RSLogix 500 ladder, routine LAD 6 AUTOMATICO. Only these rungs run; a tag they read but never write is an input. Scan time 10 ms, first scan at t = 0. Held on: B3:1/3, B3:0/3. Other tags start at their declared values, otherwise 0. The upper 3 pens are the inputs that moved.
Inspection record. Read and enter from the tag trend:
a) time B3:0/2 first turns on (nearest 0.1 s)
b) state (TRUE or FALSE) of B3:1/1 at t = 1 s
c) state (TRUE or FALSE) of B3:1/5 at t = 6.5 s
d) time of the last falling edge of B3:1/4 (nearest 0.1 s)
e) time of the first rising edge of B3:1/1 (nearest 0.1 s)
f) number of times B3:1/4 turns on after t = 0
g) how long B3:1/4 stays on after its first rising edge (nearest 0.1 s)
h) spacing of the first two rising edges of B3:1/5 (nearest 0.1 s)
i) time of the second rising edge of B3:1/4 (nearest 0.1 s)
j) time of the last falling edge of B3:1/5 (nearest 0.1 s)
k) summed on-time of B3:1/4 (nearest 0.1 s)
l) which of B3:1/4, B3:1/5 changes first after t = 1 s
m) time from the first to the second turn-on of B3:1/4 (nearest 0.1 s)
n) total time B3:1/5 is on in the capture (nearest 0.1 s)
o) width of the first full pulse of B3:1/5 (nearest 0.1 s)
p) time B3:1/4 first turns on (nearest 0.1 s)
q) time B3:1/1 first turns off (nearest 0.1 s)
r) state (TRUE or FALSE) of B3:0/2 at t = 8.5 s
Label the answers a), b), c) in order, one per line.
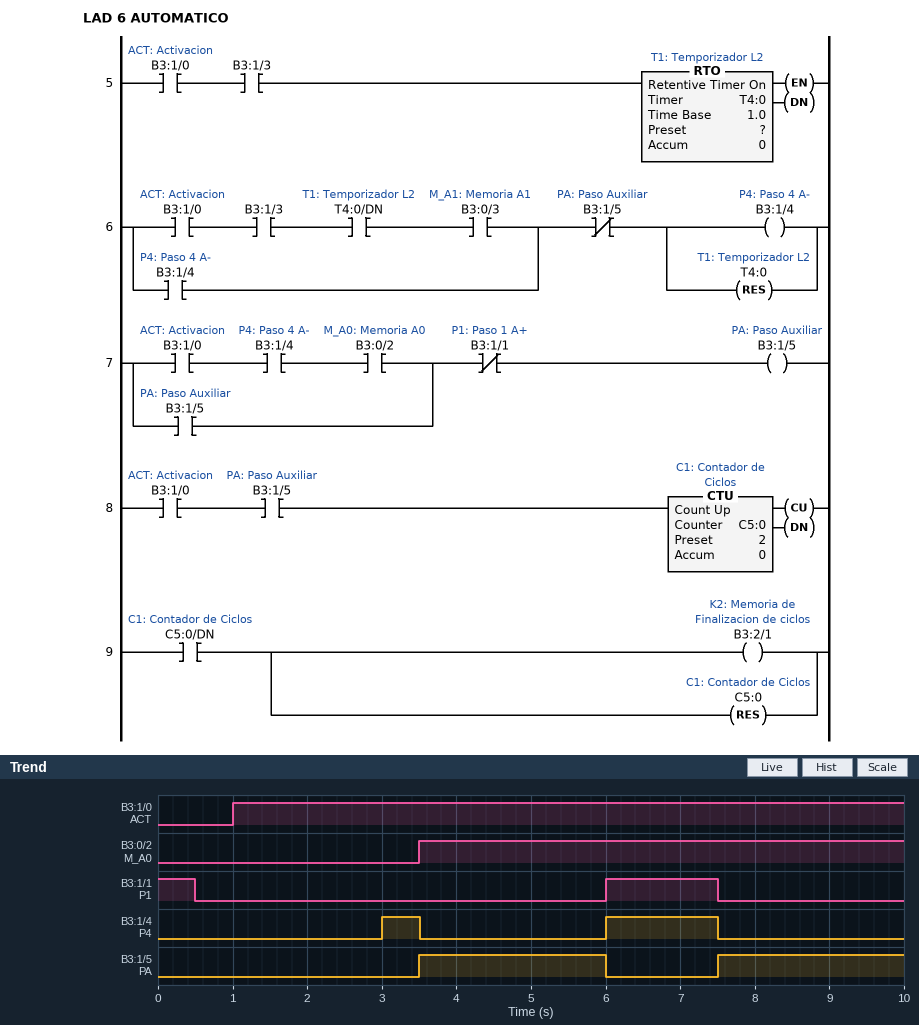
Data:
a) 3.5 s
b) FALSE
c) FALSE
d) 7.5 s
e) 6.0 s
f) 2
g) 0.5 s
h) 4.0 s
i) 6.0 s
j) 6.0 s
k) 2.0 s
l) B3:1/4
m) 3.0 s
n) 5.0 s
o) 2.5 s
p) 3.0 s
q) 0.5 s
r) TRUE
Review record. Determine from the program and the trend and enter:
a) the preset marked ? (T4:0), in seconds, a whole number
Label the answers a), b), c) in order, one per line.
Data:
a) 2 s
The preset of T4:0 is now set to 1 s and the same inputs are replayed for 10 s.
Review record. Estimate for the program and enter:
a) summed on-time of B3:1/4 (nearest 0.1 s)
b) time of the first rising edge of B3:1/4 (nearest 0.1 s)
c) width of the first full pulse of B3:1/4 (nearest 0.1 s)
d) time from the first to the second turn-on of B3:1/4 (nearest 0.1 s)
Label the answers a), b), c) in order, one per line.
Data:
a) 3.0 s
b) 2.0 s
c) 1.5 s
d) 4.0 s
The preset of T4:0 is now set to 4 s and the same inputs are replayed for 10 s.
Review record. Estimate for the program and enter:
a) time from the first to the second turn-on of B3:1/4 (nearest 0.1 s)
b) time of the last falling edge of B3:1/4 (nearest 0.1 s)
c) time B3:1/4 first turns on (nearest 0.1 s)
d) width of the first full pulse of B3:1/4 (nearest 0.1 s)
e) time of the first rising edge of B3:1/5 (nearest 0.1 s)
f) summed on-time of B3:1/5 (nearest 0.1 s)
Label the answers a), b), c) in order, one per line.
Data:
a) 4.0 s
b) 9.0 s
c) 5.0 s
d) 0.0 s
e) 5.0 s
f) 2.0 s
